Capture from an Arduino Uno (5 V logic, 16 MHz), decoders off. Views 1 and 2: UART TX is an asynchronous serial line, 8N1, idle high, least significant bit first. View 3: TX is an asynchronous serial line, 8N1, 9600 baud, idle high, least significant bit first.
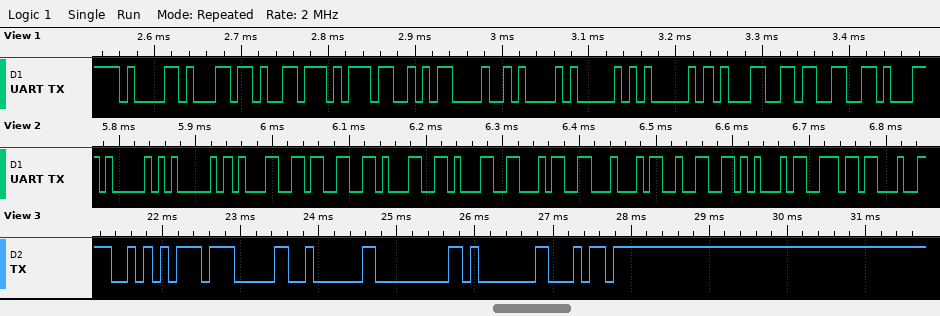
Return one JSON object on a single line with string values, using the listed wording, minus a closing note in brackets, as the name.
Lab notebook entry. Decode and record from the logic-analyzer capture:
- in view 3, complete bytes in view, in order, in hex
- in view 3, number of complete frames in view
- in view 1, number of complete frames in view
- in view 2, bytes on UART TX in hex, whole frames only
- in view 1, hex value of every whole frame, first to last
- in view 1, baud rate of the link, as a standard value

{"in view 3, complete bytes in view, in order, in hex": "AA 07 02 00 01 B4", "in view 3, number of complete frames in view": "6", "in view 1, number of complete frames in view": "10", "in view 2, bytes on UART TX in hex, whole frames only": "41 41 31 33 31 31 34 44 32 45 6E", "in view 1, hex value of every whole frame, first to last": "61 6C 76 37 0D 0A 41 41 31 33", "in view 1, baud rate of the link, as a standard value": "115200 baud"}
